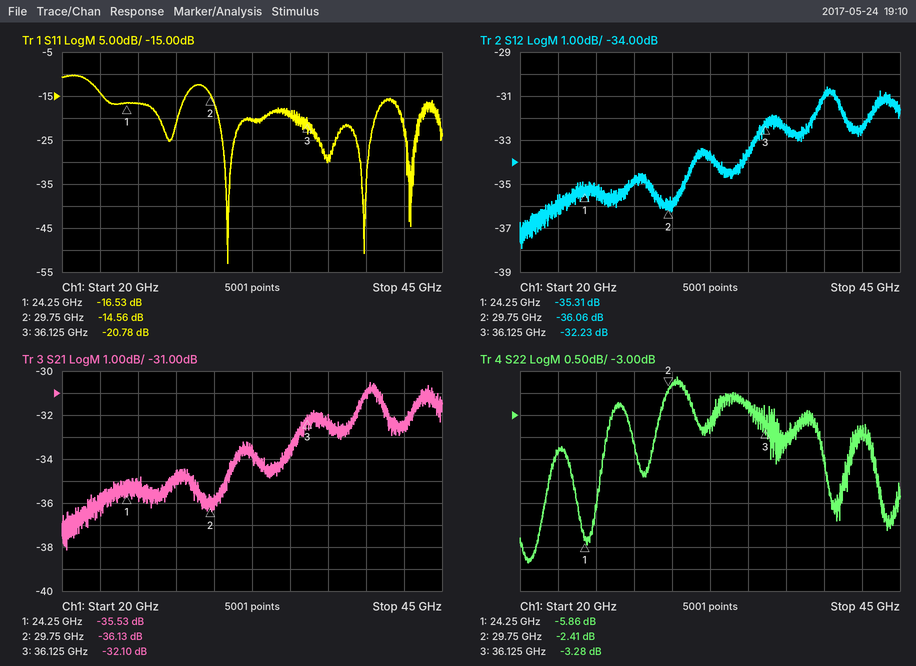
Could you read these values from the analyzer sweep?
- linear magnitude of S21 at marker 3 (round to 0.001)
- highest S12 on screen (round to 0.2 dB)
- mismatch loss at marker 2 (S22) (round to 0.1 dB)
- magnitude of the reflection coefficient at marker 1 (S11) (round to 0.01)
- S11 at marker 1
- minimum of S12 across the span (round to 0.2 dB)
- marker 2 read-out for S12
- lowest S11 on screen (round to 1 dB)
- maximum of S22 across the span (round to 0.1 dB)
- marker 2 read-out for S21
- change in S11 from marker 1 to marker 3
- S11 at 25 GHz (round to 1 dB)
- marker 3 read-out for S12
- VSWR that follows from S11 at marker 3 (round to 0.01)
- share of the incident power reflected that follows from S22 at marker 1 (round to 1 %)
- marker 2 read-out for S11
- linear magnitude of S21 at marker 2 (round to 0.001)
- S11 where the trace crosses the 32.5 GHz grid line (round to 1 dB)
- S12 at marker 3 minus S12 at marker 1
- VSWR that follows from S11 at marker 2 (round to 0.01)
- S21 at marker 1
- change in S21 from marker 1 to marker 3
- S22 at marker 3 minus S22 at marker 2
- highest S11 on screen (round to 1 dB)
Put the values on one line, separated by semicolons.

0.025; -30.6 dB; 3.7 dB; 0.15; -16.53 dB; -38.0 dB; -36.06 dB; -53 dB; -2.1 dB; -36.13 dB; -4.25 dB; -17 dB; -32.23 dB; 1.20; 26 %; -14.56 dB; 0.016; -20 dB; 3.08 dB; 1.46; -35.53 dB; 3.43 dB; -0.87 dB; -10 dB
